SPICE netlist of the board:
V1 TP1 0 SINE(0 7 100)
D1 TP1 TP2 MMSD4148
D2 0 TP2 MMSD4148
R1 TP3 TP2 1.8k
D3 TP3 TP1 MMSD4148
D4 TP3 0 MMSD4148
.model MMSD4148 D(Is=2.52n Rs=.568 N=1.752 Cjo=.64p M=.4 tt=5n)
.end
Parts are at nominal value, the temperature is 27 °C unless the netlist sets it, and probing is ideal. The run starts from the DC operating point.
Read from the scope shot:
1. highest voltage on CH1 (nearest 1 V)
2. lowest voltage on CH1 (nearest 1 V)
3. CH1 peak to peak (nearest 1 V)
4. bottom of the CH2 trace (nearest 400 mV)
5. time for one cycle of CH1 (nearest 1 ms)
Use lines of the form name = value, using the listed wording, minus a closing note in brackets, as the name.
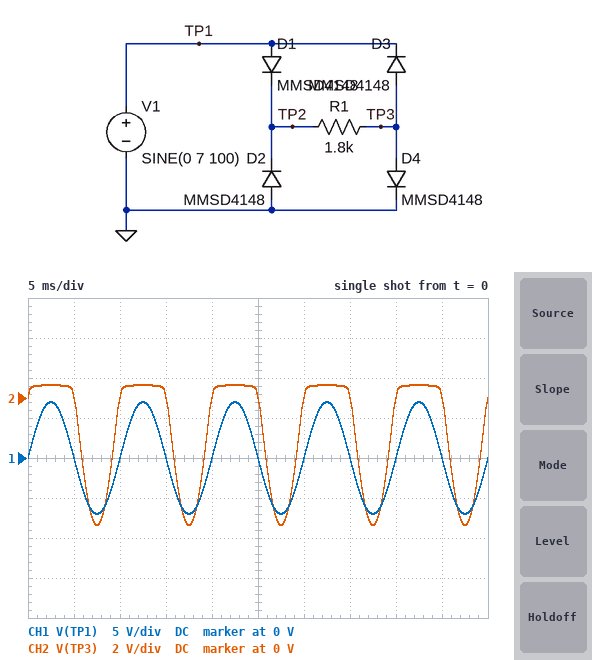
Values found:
highest voltage on CH1 = 7 V
lowest voltage on CH1 = -7 V
CH1 peak to peak = 14 V
bottom of the CH2 trace = -6.4 V
time for one cycle of CH1 = 10 ms
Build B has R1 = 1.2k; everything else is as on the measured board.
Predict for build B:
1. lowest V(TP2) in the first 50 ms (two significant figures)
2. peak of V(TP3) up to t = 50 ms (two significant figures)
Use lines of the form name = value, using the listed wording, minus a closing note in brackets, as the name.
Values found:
lowest V(TP2) in the first 50 ms = -660 mV
peak of V(TP3) up to t = 50 ms = 660 mV
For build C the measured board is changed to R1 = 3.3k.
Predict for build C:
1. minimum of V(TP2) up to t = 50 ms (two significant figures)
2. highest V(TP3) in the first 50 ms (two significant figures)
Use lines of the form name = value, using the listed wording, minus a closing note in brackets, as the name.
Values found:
minimum of V(TP2) up to t = 50 ms = -610 mV
highest V(TP3) in the first 50 ms = 610 mV
